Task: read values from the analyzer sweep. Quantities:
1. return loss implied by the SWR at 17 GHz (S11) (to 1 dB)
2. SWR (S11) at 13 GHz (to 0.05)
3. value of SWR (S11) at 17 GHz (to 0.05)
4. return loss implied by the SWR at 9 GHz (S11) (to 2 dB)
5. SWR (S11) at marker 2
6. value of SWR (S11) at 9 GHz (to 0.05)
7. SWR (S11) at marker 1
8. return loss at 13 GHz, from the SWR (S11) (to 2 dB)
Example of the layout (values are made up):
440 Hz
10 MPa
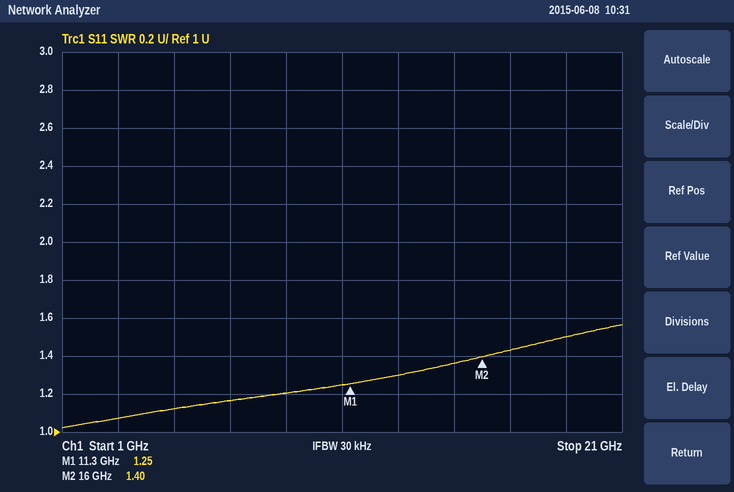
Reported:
15 dB
1.30
1.45
20 dB
1.40
1.20
1.25
18 dB
